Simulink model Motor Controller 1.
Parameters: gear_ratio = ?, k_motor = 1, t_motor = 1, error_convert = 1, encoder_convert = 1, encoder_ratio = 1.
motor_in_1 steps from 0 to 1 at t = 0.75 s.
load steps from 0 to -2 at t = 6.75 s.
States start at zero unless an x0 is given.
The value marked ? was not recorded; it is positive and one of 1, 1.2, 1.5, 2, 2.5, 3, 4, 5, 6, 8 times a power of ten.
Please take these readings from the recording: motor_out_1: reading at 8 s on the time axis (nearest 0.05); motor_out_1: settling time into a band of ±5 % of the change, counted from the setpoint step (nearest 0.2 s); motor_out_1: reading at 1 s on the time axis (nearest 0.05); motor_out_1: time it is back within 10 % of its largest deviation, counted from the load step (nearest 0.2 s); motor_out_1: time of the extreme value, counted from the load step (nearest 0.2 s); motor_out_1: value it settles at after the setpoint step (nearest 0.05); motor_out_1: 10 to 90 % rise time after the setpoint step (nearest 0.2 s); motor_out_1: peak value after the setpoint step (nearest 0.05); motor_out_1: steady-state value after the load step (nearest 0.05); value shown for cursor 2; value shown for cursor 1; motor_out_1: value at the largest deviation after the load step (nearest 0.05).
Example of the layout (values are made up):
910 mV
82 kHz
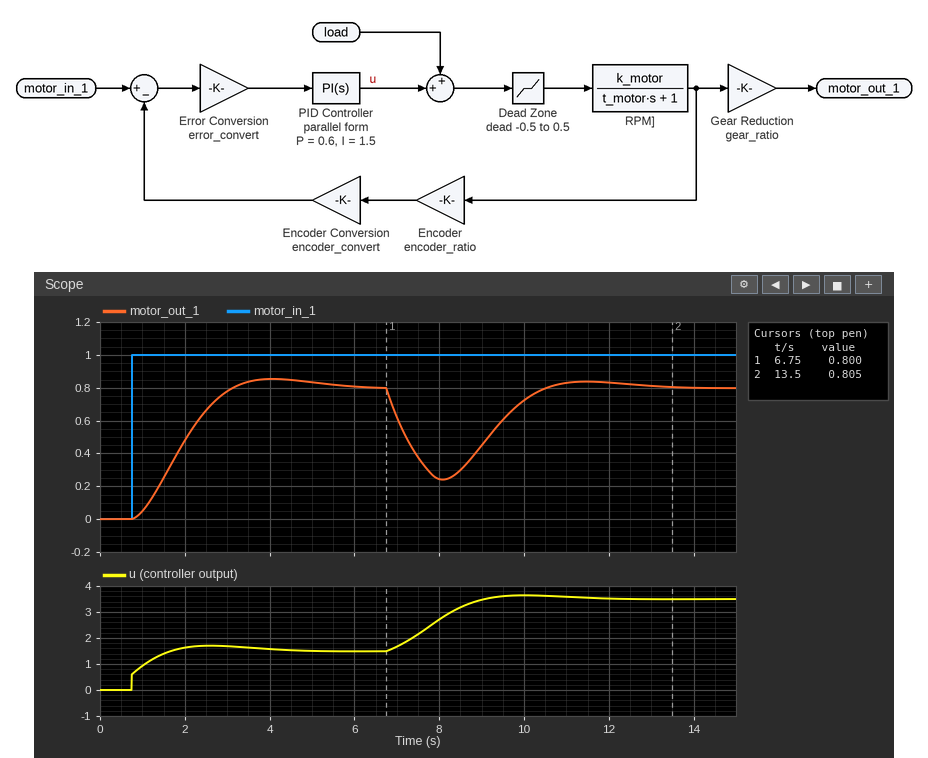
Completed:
0.25
4.0 s
0.05
3.4 s
1.4 s
0.80
1.6 s
0.85
0.80
0.805
0.800
0.25
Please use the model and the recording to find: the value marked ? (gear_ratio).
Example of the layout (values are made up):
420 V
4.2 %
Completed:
0.8
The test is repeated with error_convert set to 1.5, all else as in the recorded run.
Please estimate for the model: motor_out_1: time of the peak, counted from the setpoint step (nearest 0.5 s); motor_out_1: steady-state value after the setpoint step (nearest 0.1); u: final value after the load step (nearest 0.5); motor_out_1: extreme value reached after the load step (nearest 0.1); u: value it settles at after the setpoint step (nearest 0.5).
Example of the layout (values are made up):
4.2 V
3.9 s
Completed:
2.5 s
0.8
3.5
0.3
1.5
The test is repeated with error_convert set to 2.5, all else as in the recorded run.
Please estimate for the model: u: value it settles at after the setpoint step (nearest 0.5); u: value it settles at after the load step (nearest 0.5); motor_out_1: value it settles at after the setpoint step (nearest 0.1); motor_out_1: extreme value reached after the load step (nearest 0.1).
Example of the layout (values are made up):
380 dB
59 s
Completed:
1.5
3.5
0.8
0.4
